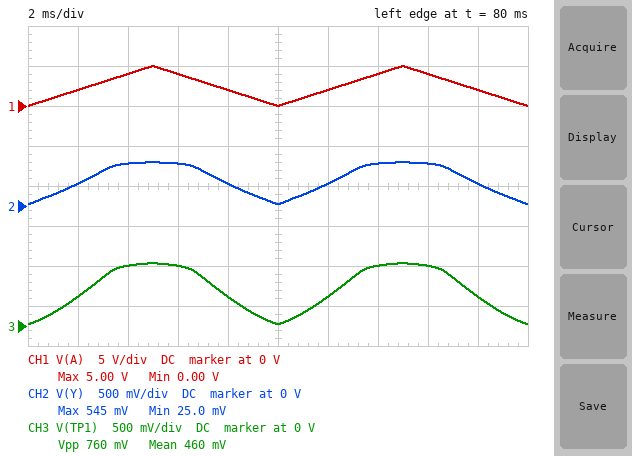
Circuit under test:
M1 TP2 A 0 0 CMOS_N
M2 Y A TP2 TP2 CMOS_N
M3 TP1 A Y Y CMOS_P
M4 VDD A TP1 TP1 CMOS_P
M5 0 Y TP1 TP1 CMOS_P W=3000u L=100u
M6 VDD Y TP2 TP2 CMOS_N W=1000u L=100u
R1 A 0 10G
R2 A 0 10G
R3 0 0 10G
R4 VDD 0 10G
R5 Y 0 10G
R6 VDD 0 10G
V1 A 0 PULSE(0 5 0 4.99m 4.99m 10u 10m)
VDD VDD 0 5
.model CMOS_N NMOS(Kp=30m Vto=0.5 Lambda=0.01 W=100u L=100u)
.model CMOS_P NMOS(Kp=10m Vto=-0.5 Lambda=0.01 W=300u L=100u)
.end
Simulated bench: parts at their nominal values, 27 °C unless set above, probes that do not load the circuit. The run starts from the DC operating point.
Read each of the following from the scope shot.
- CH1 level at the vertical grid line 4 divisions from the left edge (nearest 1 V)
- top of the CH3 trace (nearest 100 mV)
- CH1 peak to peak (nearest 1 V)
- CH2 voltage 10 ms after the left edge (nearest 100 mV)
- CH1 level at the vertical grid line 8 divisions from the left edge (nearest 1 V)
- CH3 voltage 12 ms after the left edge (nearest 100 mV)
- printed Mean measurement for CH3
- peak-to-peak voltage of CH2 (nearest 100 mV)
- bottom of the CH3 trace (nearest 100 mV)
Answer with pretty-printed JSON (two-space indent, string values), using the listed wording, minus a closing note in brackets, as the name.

{
  "CH1 level at the vertical grid line 4 divisions from the left edge": "2 V",
  "top of the CH3 trace": "800 mV",
  "CH1 peak to peak": "5 V",
  "CH2 voltage 10 ms after the left edge": "0 V",
  "CH1 level at the vertical grid line 8 divisions from the left edge": "4 V",
  "CH3 voltage 12 ms after the left edge": "400 mV",
  "printed Mean measurement for CH3": "460 mV",
  "peak-to-peak voltage of CH2": "500 mV",
  "bottom of the CH3 trace": "0 V"
}
